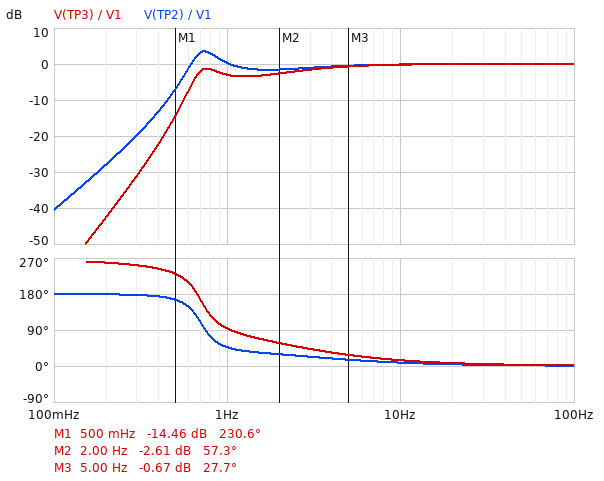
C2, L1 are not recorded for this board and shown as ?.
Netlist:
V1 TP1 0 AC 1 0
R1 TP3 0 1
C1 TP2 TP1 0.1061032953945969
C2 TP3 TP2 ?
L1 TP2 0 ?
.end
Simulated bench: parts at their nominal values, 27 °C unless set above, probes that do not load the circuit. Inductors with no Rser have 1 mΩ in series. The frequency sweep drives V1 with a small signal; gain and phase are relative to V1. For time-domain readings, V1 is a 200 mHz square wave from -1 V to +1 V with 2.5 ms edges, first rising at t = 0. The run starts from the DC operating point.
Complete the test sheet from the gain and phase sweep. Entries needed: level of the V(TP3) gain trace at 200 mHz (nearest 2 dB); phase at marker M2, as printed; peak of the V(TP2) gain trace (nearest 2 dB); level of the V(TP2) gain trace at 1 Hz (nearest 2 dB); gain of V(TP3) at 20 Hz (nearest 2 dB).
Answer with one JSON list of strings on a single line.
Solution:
["-42 dB", "57.3 deg", "4 dB", "0 dB", "0 dB"]
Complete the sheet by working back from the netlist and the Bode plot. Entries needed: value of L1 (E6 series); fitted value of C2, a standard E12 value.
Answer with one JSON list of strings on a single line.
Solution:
["220 mH", "150 mF"]
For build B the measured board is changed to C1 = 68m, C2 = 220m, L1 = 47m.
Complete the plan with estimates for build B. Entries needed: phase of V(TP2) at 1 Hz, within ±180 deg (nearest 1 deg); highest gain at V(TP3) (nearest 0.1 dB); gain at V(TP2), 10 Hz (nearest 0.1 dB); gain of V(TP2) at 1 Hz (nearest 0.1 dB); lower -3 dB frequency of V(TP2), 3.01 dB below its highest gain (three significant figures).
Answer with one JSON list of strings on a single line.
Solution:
["165 deg", "1.8 dB", "0.3 dB", "-15.6 dB", "2.07 Hz"]
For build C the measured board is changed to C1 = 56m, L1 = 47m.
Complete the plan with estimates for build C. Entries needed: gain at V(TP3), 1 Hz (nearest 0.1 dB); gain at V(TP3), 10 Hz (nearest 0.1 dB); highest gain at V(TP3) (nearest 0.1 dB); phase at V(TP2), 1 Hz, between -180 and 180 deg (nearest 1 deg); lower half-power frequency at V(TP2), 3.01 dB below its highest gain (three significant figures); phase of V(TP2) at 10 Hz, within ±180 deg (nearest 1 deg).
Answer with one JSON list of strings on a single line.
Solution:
["-20.6 dB", "0.2 dB", "0.9 dB", "169 deg", "2.13 Hz", "17 deg"]
